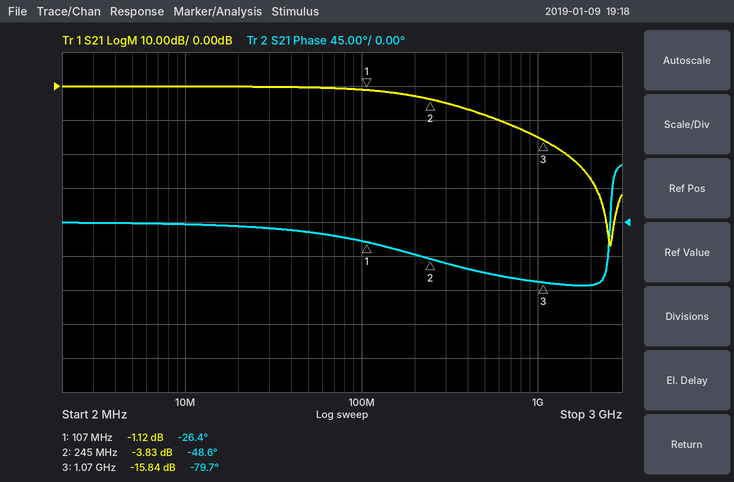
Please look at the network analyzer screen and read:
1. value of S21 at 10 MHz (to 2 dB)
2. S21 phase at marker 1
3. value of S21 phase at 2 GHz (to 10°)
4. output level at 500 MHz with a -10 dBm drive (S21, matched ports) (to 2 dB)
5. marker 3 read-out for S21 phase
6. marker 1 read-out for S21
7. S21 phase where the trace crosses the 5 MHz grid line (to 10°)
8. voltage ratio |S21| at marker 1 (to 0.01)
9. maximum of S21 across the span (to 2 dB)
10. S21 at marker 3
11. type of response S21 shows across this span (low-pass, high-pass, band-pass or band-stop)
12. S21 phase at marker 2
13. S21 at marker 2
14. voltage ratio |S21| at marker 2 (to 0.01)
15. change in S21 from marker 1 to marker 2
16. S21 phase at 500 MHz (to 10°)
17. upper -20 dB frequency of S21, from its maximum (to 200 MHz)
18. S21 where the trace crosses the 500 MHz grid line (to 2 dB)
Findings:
0 dB
-26.4°
-80°
-18 dBm
-79.7°
-1.12 dB
0°
0.88
0 dB
-15.84 dB
low-pass
-48.6°
-3.83 dB
0.64
-2.71 dB
-70°
1.4 GHz
-8 dB
